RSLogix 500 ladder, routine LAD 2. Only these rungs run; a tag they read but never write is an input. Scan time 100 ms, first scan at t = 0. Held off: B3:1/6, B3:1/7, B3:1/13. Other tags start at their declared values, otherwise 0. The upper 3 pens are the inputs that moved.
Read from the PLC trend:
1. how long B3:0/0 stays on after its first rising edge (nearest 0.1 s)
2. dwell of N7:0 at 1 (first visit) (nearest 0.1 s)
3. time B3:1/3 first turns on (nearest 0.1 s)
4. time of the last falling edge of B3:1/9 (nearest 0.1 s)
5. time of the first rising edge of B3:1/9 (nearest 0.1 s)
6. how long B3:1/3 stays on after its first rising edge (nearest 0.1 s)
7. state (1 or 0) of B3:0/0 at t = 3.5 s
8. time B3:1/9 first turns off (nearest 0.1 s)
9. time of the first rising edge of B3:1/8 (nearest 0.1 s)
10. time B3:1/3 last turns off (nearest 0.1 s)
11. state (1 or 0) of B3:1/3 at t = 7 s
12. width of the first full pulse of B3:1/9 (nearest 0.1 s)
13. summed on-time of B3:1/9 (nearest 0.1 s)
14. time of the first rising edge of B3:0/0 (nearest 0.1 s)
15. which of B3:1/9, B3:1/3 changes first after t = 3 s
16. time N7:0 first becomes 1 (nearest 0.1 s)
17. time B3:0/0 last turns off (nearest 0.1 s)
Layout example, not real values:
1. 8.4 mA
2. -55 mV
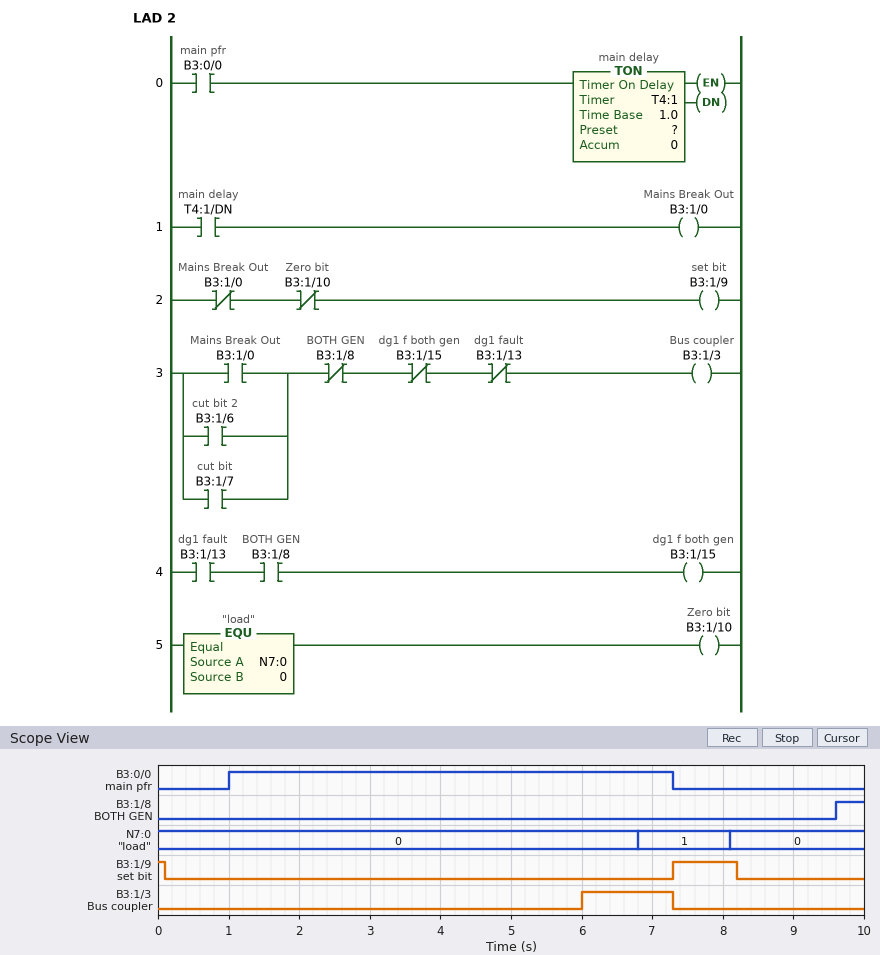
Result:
1. 6.3 s
2. 1.3 s
3. 6.0 s
4. 8.2 s
5. 7.3 s
6. 1.3 s
7. 1
8. 0.1 s
9. 9.6 s
10. 7.3 s
11. 1
12. 0.9 s
13. 1.0 s
14. 1.0 s
15. B3:1/3
16. 6.8 s
17. 7.3 s
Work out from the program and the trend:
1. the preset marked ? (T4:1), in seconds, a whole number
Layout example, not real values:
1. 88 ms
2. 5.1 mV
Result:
1. 5 s
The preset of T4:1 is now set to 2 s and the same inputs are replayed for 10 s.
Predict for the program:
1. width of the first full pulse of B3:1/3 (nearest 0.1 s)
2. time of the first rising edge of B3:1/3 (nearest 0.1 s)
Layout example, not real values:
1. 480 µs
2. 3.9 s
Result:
1. 4.3 s
2. 3.0 s
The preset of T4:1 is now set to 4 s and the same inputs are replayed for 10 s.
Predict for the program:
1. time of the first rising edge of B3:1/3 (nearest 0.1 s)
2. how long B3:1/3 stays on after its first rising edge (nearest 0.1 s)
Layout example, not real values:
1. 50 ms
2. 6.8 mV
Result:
1. 5.0 s
2. 2.3 s
